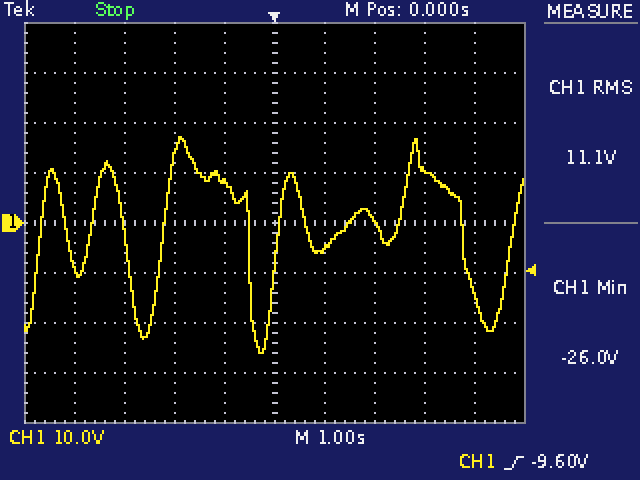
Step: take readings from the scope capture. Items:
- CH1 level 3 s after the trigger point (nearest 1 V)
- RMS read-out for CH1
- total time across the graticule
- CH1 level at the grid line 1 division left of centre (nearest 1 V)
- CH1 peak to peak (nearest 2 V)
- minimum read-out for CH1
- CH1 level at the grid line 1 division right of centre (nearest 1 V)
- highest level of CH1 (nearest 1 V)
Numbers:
11 V
11.1 V
10 s
8 V
44 V
-26.0 V
-5 V
17 V
